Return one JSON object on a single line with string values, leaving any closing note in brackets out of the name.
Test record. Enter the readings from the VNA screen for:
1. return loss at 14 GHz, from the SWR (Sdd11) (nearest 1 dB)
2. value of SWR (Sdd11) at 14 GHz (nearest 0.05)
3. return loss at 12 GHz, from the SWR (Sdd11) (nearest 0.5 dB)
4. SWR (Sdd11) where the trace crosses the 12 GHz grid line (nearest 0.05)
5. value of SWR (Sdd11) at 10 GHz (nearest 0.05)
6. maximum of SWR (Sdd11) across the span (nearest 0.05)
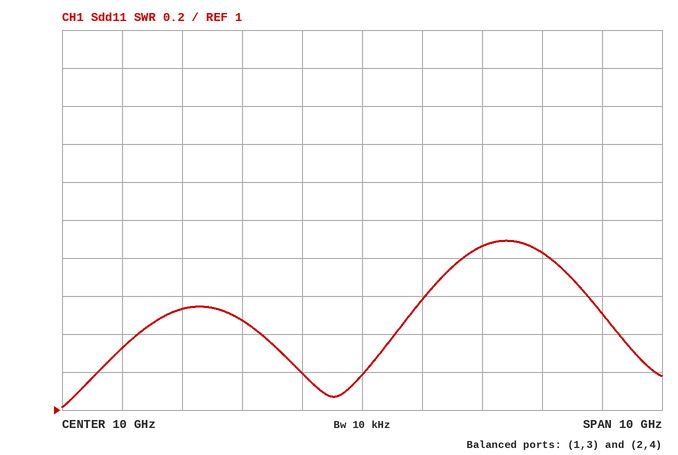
{"return loss at 14 GHz, from the SWR (Sdd11)": "14 dB", "value of SWR (Sdd11) at 14 GHz": "1.50", "return loss at 12 GHz, from the SWR (Sdd11)": "10.5 dB", "SWR (Sdd11) where the trace crosses the 12 GHz grid line": "1.85", "value of SWR (Sdd11) at 10 GHz": "1.20", "maximum of SWR (Sdd11) across the span": "1.90"}
